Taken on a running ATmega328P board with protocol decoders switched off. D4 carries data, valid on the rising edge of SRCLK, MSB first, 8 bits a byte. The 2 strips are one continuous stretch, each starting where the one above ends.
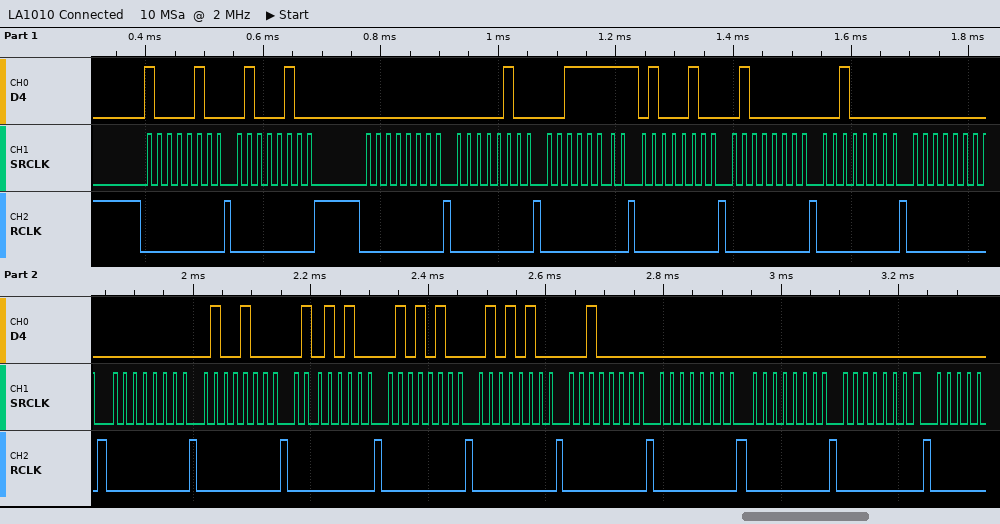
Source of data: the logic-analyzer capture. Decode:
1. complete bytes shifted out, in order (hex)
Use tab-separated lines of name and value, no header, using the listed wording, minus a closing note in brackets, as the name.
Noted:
complete bytes shifted out, in order	84 44 00 04 3F 44 40 20 00 00 48 54 54 54 20 00 00 00
